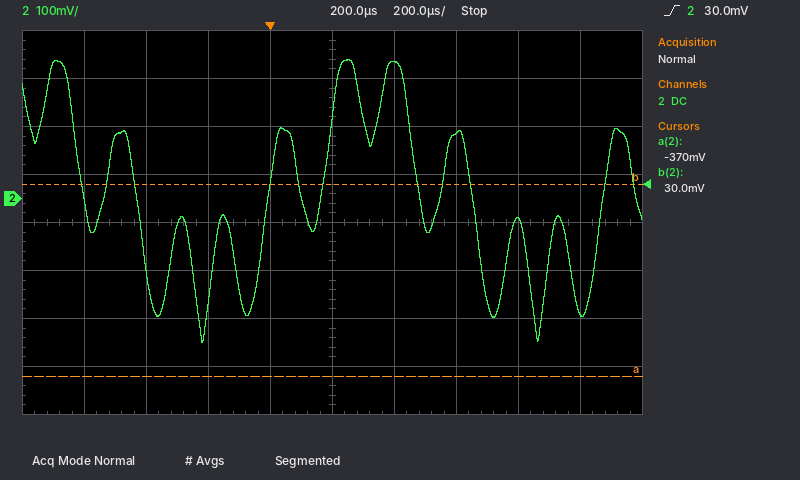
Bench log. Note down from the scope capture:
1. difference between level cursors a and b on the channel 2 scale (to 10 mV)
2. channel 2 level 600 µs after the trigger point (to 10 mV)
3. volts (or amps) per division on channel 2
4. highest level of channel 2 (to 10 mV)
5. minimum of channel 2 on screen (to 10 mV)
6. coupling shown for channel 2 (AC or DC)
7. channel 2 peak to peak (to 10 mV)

400 mV
140 mV
100 mV
290 mV
-300 mV
DC
590 mV
